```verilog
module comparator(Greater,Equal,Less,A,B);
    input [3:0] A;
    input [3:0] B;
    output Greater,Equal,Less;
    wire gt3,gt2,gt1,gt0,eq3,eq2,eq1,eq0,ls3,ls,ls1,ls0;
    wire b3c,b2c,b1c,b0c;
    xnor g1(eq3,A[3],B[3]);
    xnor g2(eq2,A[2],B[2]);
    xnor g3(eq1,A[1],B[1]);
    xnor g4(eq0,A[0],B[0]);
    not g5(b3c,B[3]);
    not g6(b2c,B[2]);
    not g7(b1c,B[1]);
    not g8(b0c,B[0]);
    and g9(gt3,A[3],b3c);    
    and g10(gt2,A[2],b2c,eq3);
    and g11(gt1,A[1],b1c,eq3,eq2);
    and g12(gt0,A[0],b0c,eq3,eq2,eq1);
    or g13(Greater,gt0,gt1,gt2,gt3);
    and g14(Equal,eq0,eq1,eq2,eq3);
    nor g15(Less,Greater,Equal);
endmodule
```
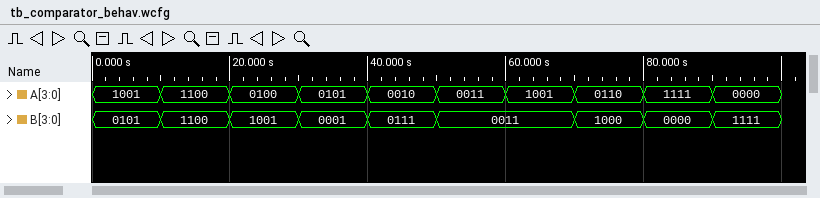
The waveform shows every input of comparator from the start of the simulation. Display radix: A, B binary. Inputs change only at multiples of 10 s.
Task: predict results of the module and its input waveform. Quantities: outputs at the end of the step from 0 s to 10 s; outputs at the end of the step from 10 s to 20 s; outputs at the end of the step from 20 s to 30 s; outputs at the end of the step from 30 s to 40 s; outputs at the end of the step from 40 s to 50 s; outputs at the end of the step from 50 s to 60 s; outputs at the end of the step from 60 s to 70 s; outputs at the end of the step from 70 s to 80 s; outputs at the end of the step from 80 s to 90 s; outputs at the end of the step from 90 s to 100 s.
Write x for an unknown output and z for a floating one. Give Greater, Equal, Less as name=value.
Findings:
Greater=1, Equal=0, Less=0
Greater=0, Equal=1, Less=0
Greater=0, Equal=0, Less=1
Greater=1, Equal=0, Less=0
Greater=0, Equal=0, Less=1
Greater=0, Equal=1, Less=0
Greater=1, Equal=0, Less=0
Greater=0, Equal=0, Less=1
Greater=1, Equal=0, Less=0
Greater=0, Equal=0, Less=1
